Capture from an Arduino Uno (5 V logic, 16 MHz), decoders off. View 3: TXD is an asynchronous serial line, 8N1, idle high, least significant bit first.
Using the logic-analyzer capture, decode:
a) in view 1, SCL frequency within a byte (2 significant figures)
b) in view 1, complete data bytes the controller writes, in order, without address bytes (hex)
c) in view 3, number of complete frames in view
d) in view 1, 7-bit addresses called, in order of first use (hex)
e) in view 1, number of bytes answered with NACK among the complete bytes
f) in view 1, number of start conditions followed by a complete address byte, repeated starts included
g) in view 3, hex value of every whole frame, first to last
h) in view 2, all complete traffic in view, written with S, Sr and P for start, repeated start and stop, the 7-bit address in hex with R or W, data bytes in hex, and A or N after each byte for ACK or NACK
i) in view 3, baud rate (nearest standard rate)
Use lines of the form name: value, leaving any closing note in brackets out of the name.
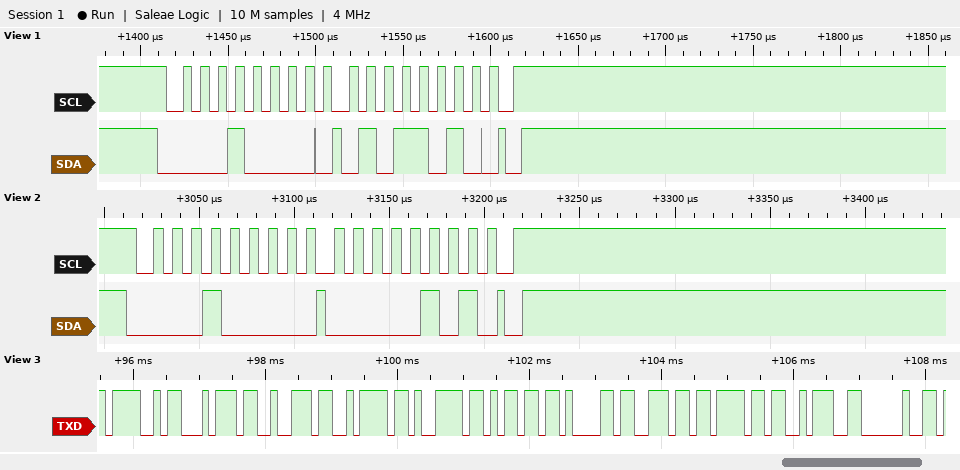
in view 1, SCL frequency within a byte: 100 kHz
in view 1, complete data bytes the controller writes, in order, without address bytes: 5A
in view 3, number of complete frames in view: 11
in view 1, 7-bit addresses called, in order of first use: 0x08
in view 1, number of bytes answered with NACK among the complete bytes: 0
in view 1, number of start conditions followed by a complete address byte, repeated starts included: 1
in view 3, hex value of every whole frame, first to last: 4F 74 72 7A 79 6D 61 6E 6F 3A 20
in view 2, all complete traffic in view, written with S, Sr and P for start, repeated start and stop, the 7-bit address in hex with R or W, data bytes in hex, and A or N after each byte for ACK or NACK: S 08W A 05 A P
in view 3, baud rate: 9600 baud
